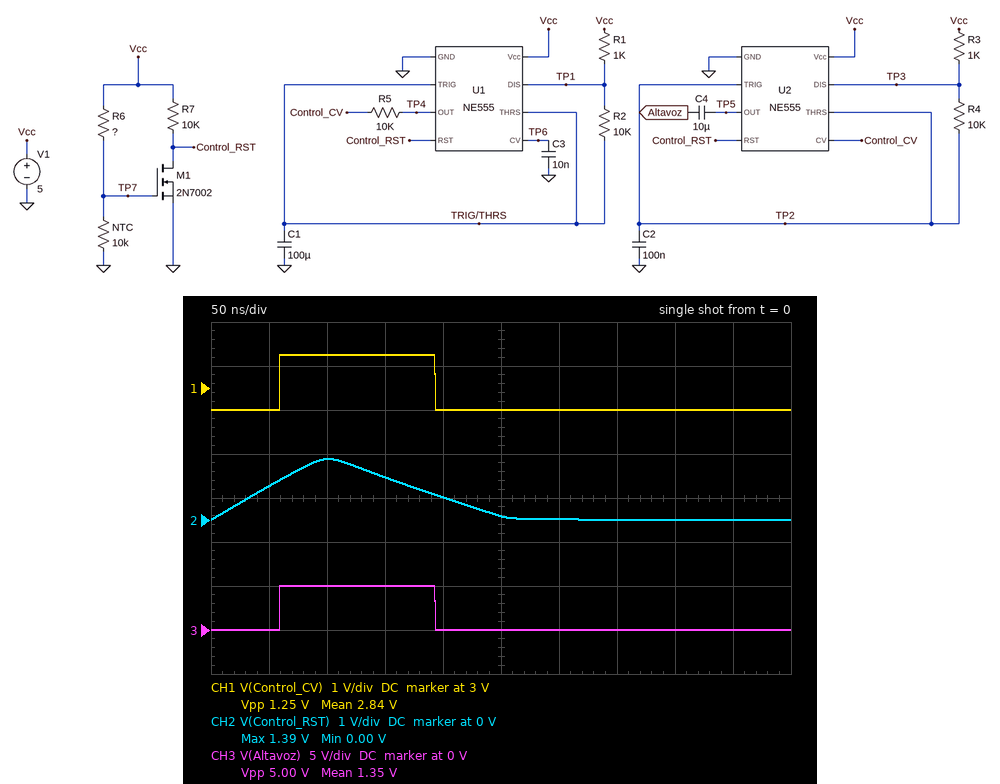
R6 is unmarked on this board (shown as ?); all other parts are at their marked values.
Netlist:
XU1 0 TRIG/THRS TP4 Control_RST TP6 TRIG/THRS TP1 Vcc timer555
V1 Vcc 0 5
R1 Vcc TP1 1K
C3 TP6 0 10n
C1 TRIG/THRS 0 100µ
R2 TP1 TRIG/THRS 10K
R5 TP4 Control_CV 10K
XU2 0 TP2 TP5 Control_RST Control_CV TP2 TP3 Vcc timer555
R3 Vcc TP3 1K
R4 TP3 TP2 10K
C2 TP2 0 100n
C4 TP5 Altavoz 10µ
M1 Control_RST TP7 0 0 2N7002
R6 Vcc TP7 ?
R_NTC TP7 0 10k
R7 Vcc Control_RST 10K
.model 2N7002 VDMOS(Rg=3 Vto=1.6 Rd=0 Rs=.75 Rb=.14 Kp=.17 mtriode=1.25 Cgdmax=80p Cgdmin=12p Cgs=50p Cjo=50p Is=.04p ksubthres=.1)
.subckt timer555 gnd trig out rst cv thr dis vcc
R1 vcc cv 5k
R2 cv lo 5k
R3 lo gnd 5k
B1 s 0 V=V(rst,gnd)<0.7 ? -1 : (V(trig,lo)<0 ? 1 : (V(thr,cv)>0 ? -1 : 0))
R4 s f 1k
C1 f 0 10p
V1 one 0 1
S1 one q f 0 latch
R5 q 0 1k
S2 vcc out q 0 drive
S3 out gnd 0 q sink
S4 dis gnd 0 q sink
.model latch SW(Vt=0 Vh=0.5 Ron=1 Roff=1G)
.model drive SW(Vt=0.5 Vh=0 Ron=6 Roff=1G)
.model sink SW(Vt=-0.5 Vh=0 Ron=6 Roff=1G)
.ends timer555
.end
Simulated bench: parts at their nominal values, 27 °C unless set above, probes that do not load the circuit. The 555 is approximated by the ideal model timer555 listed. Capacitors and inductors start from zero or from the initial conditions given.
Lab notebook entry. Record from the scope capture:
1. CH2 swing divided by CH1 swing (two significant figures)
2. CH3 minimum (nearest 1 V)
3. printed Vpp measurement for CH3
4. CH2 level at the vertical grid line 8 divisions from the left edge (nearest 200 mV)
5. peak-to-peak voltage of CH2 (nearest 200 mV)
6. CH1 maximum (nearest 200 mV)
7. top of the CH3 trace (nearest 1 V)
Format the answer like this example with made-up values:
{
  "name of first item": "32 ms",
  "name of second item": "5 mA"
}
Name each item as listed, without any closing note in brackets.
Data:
{
  "CH2 swing divided by CH1 swing": "1.1",
  "CH3 minimum": "0 V",
  "printed Vpp measurement for CH3": "5.00 V",
  "CH2 level at the vertical grid line 8 divisions from the left edge": "0 V",
  "peak-to-peak voltage of CH2": "1.4 V",
  "CH1 maximum": "3.8 V",
  "top of the CH3 trace": "5 V"
}
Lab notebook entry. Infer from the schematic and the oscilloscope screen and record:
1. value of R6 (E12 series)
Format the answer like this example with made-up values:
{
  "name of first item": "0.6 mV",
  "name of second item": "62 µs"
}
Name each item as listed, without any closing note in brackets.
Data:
{
  "value of R6": "3.9 kΩ"
}
